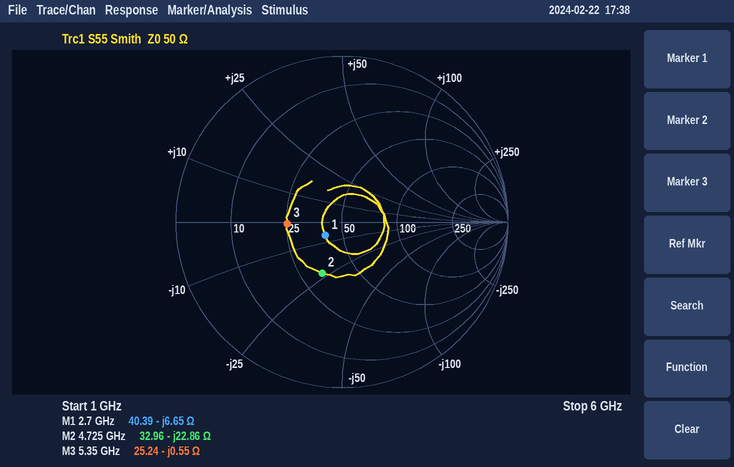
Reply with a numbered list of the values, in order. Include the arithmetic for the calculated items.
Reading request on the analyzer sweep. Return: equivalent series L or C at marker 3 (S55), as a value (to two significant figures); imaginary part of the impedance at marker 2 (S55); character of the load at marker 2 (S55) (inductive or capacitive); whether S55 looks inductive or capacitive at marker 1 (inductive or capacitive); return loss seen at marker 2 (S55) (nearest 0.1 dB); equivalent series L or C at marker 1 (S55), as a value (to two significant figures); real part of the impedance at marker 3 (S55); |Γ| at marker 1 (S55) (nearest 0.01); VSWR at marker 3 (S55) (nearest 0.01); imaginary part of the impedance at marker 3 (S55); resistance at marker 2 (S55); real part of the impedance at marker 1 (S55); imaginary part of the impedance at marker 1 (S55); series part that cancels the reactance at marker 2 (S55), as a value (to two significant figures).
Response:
1. C = 1/(2π × 5.35 GHz × 0.55 Ω) ≈ 54 pF
2. -22.86 Ω
3. capacitive
4. capacitive
5. 9.6 dB
6. C = 1/(2π × 2.7 GHz × 6.65 Ω) ≈ 8.9 pF
7. 25.24 Ω
8. 0.13
9. 1.98
10. -0.55 Ω
11. 32.96 Ω
12. 40.39 Ω
13. -6.65 Ω
14. L = 22.86 Ω/(2π × 4.725 GHz) ≈ 770 pH
